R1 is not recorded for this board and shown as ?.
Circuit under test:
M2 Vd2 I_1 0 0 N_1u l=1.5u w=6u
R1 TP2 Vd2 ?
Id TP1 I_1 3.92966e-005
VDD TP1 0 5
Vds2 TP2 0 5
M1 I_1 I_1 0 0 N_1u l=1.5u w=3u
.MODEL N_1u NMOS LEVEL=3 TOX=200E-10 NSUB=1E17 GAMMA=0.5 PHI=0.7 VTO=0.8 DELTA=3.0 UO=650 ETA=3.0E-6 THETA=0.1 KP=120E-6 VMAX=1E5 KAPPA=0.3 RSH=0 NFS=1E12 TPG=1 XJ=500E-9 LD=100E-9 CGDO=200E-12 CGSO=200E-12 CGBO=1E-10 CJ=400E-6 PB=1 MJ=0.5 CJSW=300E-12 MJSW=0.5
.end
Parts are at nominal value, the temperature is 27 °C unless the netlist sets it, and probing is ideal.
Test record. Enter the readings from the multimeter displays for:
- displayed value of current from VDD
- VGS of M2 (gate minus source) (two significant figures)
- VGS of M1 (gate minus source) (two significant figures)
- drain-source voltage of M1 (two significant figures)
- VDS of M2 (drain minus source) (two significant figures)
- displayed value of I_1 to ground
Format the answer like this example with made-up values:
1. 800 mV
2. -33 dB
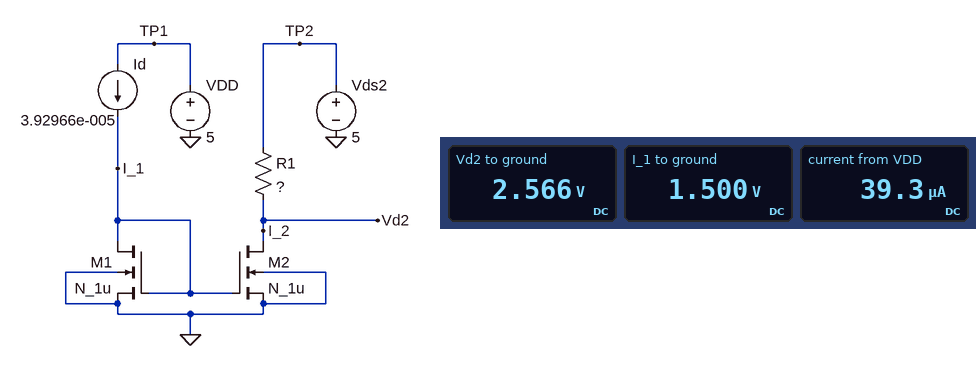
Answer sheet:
1. 39.3 µA
2. 1.5 V
3. 1.5 V
4. 1.5 V
5. 2.6 V
6. 1.500 V
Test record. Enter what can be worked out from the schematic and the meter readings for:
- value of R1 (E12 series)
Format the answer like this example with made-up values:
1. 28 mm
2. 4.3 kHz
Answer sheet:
1. 27 kΩ
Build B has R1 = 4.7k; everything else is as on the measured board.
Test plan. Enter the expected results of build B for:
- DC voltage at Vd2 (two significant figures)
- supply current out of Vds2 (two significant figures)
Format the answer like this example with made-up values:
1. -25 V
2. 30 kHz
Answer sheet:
1. 4.6 V
2. 93 µA
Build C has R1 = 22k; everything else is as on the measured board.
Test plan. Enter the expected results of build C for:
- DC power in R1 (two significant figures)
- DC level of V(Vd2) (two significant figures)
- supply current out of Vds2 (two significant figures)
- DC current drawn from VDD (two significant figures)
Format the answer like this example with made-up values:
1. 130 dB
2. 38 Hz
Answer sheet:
1. 180 µW
2. 3.0 V
3. 91 µA
4. 39 µA
